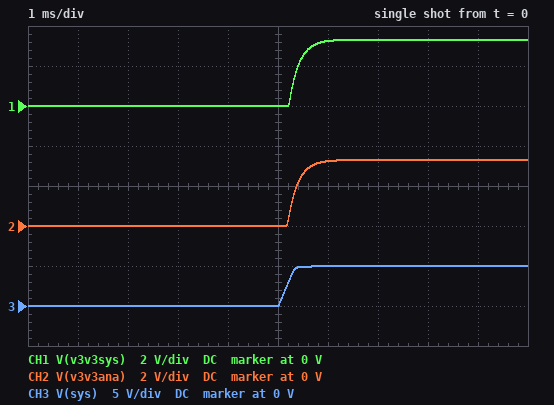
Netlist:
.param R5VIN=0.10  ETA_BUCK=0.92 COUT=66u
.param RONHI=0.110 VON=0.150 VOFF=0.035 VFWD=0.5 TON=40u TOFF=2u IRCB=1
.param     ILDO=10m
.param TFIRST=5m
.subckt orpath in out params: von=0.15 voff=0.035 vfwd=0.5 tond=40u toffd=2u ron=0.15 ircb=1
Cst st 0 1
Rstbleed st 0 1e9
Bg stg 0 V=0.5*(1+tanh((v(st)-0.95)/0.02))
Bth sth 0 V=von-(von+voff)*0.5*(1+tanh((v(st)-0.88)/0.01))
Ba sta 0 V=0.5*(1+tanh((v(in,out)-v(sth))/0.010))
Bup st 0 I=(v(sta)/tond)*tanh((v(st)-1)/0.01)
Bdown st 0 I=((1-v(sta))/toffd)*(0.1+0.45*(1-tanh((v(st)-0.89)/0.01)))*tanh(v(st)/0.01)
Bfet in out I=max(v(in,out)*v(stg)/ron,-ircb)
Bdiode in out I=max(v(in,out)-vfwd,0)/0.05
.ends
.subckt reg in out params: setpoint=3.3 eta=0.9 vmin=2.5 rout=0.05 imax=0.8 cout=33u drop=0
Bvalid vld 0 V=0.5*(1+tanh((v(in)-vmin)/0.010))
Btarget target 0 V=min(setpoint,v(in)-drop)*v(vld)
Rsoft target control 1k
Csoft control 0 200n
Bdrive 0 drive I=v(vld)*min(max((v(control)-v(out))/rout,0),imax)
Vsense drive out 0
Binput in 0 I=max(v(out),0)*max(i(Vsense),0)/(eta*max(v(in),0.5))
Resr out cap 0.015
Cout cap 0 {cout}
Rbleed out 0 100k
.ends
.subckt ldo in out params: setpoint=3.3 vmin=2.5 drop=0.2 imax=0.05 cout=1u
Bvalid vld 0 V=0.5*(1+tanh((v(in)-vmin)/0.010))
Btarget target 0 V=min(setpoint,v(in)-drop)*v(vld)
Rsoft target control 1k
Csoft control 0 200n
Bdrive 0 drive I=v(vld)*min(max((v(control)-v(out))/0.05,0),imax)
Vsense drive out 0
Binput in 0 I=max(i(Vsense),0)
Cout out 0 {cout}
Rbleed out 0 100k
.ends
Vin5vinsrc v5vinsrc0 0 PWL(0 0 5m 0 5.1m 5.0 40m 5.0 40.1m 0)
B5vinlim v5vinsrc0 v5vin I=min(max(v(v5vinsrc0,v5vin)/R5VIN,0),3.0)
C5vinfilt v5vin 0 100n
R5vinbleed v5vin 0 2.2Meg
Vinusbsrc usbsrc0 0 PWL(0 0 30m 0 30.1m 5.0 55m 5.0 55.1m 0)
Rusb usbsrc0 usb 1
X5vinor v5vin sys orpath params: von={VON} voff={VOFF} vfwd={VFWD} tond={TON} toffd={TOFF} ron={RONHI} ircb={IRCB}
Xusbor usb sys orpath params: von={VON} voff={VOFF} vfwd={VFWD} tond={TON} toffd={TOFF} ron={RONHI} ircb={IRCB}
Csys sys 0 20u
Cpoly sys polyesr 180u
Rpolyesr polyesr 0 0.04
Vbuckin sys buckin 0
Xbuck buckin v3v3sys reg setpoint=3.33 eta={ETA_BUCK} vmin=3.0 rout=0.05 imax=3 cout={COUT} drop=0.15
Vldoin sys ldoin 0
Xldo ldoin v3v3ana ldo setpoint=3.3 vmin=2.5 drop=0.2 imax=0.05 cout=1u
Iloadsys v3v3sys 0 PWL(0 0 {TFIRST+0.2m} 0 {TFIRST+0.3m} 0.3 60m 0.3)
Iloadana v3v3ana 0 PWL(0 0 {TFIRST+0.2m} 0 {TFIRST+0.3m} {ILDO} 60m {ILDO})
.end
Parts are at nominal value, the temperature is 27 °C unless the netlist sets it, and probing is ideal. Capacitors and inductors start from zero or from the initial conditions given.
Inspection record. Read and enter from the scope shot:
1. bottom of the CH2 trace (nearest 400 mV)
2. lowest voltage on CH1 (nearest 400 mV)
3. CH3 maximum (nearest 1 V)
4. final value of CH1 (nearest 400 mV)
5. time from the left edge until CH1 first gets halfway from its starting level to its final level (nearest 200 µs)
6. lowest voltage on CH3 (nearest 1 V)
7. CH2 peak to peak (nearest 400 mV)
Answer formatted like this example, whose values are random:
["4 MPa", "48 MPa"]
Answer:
["0 V", "0 V", "5 V", "3.2 V", "5.4 ms", "0 V", "3.2 V"]
